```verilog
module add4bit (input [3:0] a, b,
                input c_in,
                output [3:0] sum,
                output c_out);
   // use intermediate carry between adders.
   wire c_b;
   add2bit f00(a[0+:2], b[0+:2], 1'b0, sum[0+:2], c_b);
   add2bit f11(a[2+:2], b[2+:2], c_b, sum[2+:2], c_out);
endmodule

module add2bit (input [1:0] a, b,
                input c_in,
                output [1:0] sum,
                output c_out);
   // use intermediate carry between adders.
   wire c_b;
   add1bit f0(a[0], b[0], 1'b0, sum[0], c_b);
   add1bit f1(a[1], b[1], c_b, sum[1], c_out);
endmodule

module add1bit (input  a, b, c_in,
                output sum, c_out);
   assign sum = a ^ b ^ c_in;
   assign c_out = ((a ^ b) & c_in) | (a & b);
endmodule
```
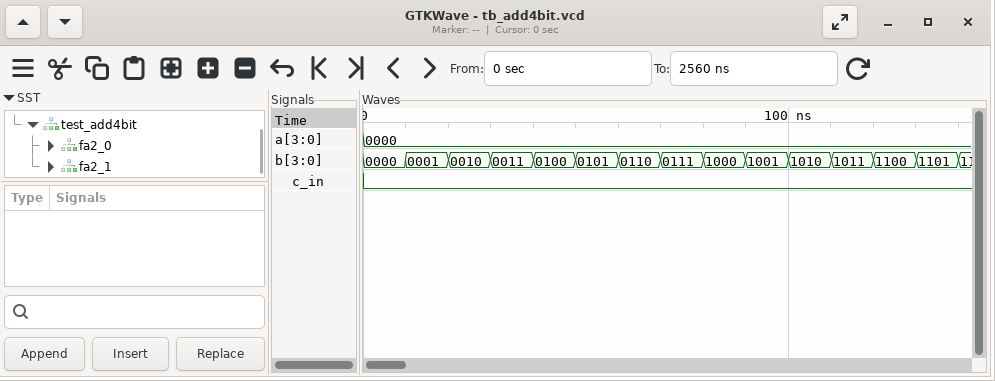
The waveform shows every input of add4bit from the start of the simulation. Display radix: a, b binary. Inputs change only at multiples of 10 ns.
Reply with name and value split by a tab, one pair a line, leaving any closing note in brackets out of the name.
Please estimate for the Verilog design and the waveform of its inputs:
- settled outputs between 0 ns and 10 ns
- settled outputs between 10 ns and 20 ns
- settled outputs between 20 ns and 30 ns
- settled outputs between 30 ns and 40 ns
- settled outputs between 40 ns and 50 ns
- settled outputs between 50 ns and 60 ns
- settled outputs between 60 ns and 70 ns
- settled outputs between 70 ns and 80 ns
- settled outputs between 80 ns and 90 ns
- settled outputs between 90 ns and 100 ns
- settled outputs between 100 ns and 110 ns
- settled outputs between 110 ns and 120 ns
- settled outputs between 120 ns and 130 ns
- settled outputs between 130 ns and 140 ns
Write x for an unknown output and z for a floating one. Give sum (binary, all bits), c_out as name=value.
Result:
settled outputs between 0 ns and 10 ns	sum=0000, c_out=0
settled outputs between 10 ns and 20 ns	sum=0001, c_out=0
settled outputs between 20 ns and 30 ns	sum=0010, c_out=0
settled outputs between 30 ns and 40 ns	sum=0011, c_out=0
settled outputs between 40 ns and 50 ns	sum=0100, c_out=0
settled outputs between 50 ns and 60 ns	sum=0101, c_out=0
settled outputs between 60 ns and 70 ns	sum=0110, c_out=0
settled outputs between 70 ns and 80 ns	sum=0111, c_out=0
settled outputs between 80 ns and 90 ns	sum=1000, c_out=0
settled outputs between 90 ns and 100 ns	sum=1001, c_out=0
settled outputs between 100 ns and 110 ns	sum=1010, c_out=0
settled outputs between 110 ns and 120 ns	sum=1011, c_out=0
settled outputs between 120 ns and 130 ns	sum=1100, c_out=0
settled outputs between 130 ns and 140 ns	sum=1101, c_out=0
